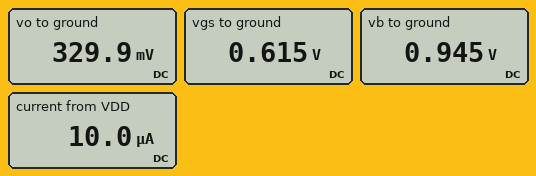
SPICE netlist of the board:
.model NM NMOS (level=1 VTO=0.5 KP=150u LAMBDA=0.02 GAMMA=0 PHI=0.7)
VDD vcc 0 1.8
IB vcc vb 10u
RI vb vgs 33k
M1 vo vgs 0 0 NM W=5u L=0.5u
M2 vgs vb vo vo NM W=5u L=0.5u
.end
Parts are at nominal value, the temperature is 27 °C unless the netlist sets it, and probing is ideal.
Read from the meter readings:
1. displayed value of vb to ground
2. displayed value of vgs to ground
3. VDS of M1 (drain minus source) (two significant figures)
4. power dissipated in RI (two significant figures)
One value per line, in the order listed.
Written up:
0.945 V
0.615 V
330 mV
3.3 µW
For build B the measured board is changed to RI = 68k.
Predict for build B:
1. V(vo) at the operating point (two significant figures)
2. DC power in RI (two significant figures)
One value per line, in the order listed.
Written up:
580 mV
6.8 µW
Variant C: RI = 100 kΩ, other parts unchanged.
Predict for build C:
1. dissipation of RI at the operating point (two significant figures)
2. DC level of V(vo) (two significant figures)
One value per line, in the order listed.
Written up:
10 µW
600 mV
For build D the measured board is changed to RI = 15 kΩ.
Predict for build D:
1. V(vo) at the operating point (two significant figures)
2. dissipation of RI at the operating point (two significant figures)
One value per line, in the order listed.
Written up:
150 mV
1.5 µW
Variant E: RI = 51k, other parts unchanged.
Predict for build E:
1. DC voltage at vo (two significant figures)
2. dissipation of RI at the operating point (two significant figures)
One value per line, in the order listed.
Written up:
510 mV
5.1 µW
